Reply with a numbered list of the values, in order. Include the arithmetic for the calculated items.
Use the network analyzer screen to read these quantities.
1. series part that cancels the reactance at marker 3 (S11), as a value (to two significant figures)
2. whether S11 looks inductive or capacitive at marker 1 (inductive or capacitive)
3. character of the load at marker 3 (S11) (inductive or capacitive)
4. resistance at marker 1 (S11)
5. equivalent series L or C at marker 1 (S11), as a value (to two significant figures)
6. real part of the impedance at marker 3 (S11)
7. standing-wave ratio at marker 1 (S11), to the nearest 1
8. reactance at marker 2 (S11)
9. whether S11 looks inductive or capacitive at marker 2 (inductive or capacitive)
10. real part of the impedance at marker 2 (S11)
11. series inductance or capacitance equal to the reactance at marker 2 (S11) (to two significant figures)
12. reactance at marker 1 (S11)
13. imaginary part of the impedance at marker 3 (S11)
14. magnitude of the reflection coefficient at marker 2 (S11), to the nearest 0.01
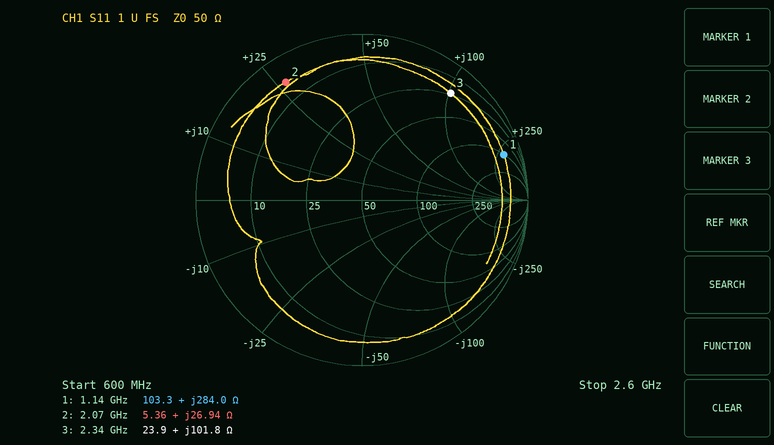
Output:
1. C = 1/(2π × 2.34 GHz × 101.8 Ω) ≈ 668 fF, so 670 fF to two significant figures
2. inductive
3. inductive
4. 103.3 Ω
5. L = 284 Ω/(2π × 1.14 GHz) ≈ 40 nH
6. 23.9 Ω
7. 18
8. +26.94 Ω
9. inductive
10. 5.36 Ω
11. L = 26.94 Ω/(2π × 2.07 GHz) ≈ 2.1 nH
12. +284.0 Ω
13. +101.8 Ω
14. 0.85
